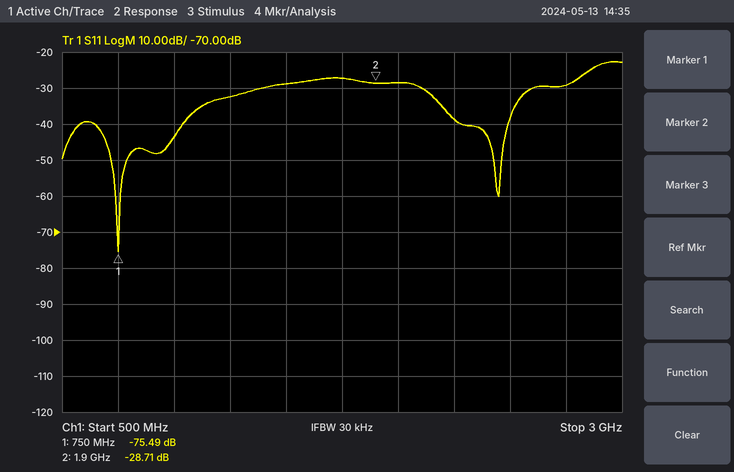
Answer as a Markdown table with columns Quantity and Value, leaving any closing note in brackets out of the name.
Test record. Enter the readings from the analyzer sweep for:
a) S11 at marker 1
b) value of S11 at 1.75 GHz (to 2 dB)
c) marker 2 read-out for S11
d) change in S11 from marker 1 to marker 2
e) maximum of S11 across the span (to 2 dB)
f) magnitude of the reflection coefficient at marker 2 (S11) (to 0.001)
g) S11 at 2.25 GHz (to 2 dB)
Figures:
| Quantity | Value |
|---|---|
| S11 at marker 1 | -75.49 dB |
| value of S11 at 1.75 GHz | -28 dB |
| marker 2 read-out for S11 | -28.71 dB |
| change in S11 from marker 1 to marker 2 | 46.78 dB |
| maximum of S11 across the span | -22 dB |
| magnitude of the reflection coefficient at marker 2 (S11) | 0.037 |
| S11 at 2.25 GHz | -38 dB |
